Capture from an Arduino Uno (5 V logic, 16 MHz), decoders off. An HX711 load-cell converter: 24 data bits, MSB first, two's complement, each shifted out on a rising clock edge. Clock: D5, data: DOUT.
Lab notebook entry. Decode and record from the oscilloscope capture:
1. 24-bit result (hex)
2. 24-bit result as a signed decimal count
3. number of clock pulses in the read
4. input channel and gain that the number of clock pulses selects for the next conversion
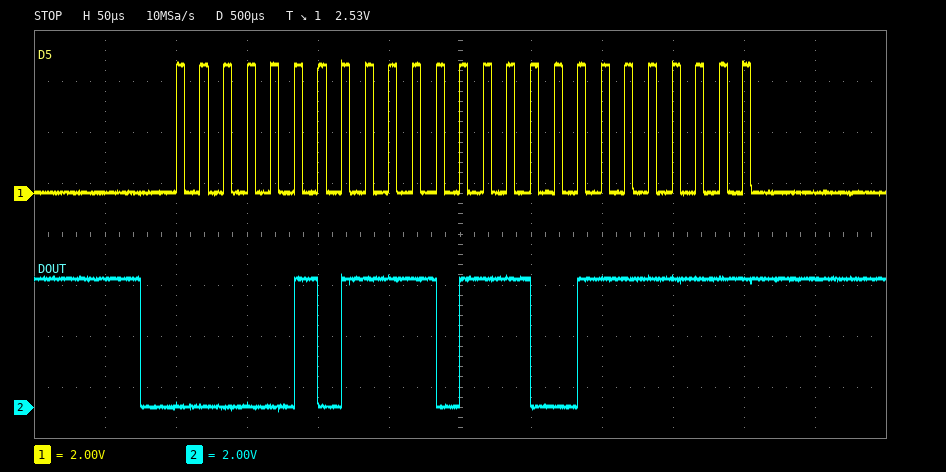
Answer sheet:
0x05EE7F
388735
25
channel A, gain 128
